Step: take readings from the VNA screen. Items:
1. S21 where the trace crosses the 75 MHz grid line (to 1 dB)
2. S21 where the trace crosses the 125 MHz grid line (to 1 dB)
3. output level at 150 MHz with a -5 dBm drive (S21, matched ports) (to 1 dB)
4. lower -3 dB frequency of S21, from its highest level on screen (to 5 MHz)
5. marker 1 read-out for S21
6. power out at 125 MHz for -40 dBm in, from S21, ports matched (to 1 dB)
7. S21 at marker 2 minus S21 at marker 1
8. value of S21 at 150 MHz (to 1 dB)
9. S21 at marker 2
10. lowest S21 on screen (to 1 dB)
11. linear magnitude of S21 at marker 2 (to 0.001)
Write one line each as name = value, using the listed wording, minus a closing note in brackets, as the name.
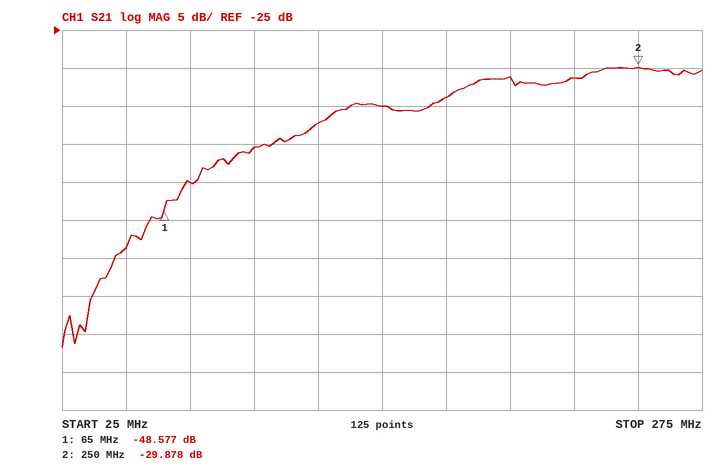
S21 where the trace crosses the 75 MHz grid line = -45 dB
S21 where the trace crosses the 125 MHz grid line = -37 dB
output level at 150 MHz with a -5 dBm drive (S21, matched ports) = -40 dBm
lower -3 dB frequency of S21, from its highest level on screen = 180 MHz
marker 1 read-out for S21 = -48.577 dB
power out at 125 MHz for -40 dBm in, from S21, ports matched = -77 dBm
S21 at marker 2 minus S21 at marker 1 = 18.699 dB
value of S21 at 150 MHz = -35 dB
S21 at marker 2 = -29.878 dB
lowest S21 on screen = -67 dB
linear magnitude of S21 at marker 2 = 0.032
